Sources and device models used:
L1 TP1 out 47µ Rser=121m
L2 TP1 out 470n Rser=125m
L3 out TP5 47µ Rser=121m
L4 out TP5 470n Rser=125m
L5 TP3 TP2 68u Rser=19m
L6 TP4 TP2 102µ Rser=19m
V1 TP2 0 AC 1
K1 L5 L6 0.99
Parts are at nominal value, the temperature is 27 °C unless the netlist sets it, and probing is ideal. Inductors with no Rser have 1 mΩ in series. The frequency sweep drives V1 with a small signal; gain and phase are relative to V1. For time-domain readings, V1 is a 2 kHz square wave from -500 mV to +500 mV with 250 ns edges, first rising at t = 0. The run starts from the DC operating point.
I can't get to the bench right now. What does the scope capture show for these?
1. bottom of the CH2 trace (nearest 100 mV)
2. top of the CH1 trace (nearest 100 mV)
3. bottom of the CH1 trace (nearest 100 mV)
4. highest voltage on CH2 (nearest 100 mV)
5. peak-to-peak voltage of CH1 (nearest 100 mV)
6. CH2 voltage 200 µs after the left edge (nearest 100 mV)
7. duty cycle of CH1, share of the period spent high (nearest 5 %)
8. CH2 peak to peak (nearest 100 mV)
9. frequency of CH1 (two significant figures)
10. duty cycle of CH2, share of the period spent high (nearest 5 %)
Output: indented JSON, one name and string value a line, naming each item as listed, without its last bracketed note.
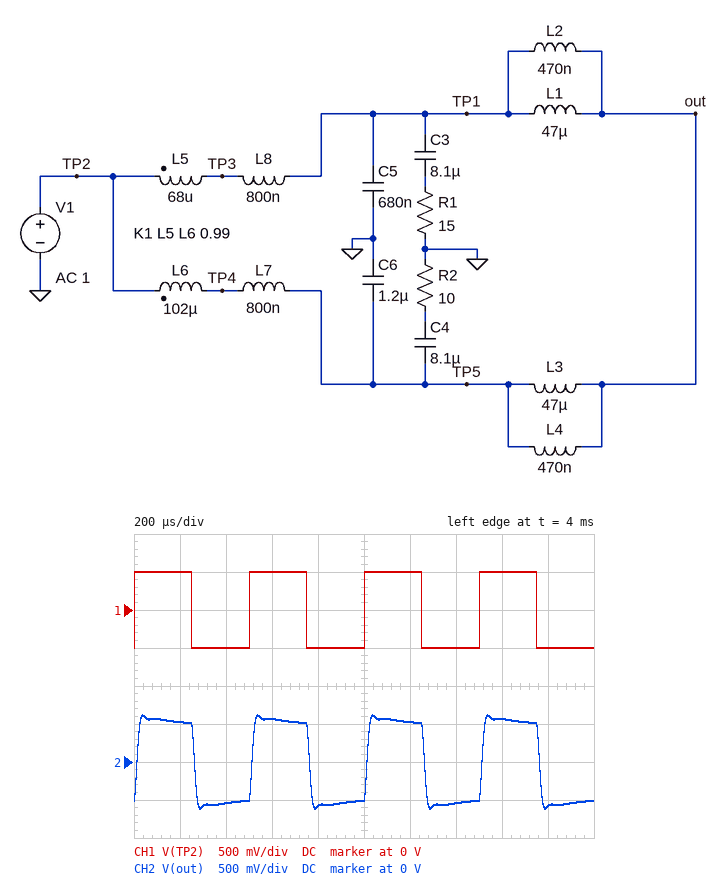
{
  "bottom of the CH2 trace": "-600 mV",
  "top of the CH1 trace": "500 mV",
  "bottom of the CH1 trace": "-500 mV",
  "highest voltage on CH2": "600 mV",
  "peak-to-peak voltage of CH1": "1.0 V",
  "CH2 voltage 200 µs after the left edge": "500 mV",
  "duty cycle of CH1, share of the period spent high": "50 %",
  "CH2 peak to peak": "1.2 V",
  "frequency of CH1": "2.0 kHz",
  "duty cycle of CH2, share of the period spent high": "50 %"
}
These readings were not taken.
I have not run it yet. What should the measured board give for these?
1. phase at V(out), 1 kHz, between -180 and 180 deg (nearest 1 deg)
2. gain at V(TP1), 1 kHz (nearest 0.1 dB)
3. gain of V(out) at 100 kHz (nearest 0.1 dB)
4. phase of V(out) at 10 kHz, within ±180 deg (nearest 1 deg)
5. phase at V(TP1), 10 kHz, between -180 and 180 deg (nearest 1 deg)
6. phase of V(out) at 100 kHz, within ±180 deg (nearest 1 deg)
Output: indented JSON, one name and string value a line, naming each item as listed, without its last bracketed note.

{
  "phase at V(out), 1 kHz, between -180 and 180 deg": "-2 deg",
  "gain at V(TP1), 1 kHz": "0.3 dB",
  "gain of V(out) at 100 kHz": "-33.2 dB",
  "phase of V(out) at 10 kHz, within ±180 deg": "-48 deg",
  "phase at V(TP1), 10 kHz, between -180 and 180 deg": "-45 deg",
  "phase of V(out) at 100 kHz, within ±180 deg": "-157 deg"
}
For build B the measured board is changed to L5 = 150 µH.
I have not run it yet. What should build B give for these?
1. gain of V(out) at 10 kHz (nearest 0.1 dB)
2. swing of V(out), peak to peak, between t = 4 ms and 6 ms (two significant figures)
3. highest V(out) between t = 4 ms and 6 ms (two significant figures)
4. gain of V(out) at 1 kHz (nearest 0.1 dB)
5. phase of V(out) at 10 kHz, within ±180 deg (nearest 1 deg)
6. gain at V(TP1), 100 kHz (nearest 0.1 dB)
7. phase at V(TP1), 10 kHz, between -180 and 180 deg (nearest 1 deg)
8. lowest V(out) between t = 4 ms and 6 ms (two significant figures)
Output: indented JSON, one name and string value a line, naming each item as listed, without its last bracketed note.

{
  "gain of V(out) at 10 kHz": "-0.8 dB",
  "swing of V(out), peak to peak, between t = 4 ms and 6 ms": "1.2 V",
  "highest V(out) between t = 4 ms and 6 ms": "580 mV",
  "gain of V(out) at 1 kHz": "0.5 dB",
  "phase of V(out) at 10 kHz, within ±180 deg": "-61 deg",
  "gain at V(TP1), 100 kHz": "-26.6 dB",
  "phase at V(TP1), 10 kHz, between -180 and 180 deg": "-65 deg",
  "lowest V(out) between t = 4 ms and 6 ms": "-580 mV"
}
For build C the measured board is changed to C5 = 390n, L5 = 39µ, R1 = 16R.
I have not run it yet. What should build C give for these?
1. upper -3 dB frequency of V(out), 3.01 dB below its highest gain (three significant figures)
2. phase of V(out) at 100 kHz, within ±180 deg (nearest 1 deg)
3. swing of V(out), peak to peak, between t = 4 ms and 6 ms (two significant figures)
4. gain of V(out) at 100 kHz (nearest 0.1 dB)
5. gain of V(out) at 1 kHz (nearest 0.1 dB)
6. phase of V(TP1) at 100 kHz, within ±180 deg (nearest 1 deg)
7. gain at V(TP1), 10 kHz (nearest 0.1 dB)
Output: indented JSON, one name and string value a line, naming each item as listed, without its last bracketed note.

{
  "upper -3 dB frequency of V(out), 3.01 dB below its highest gain": "40.9 kHz",
  "phase of V(out) at 100 kHz, within ±180 deg": "-148 deg",
  "swing of V(out), peak to peak, between t = 4 ms and 6 ms": "1.3 V",
  "gain of V(out) at 100 kHz": "-21.6 dB",
  "gain of V(out) at 1 kHz": "0.2 dB",
  "phase of V(TP1) at 100 kHz, within ±180 deg": "-85 deg",
  "gain at V(TP1), 10 kHz": "-0.1 dB"
}
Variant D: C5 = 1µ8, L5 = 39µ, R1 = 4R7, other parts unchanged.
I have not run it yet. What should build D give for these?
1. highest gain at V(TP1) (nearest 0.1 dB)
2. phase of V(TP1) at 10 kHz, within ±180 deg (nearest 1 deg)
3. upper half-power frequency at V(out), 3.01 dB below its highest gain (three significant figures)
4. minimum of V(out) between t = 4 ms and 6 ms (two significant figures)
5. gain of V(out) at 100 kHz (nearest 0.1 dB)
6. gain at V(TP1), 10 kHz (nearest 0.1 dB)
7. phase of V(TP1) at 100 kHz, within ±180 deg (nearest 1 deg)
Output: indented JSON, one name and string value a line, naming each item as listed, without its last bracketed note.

{
  "highest gain at V(TP1)": "0.5 dB",
  "phase of V(TP1) at 10 kHz, within ±180 deg": "-24 deg",
  "upper half-power frequency at V(out), 3.01 dB below its highest gain": "31.0 kHz",
  "minimum of V(out) between t = 4 ms and 6 ms": "-590 mV",
  "gain of V(out) at 100 kHz": "-22.5 dB",
  "gain at V(TP1), 10 kHz": "0 dB",
  "phase of V(TP1) at 100 kHz, within ±180 deg": "-91 deg"
}
